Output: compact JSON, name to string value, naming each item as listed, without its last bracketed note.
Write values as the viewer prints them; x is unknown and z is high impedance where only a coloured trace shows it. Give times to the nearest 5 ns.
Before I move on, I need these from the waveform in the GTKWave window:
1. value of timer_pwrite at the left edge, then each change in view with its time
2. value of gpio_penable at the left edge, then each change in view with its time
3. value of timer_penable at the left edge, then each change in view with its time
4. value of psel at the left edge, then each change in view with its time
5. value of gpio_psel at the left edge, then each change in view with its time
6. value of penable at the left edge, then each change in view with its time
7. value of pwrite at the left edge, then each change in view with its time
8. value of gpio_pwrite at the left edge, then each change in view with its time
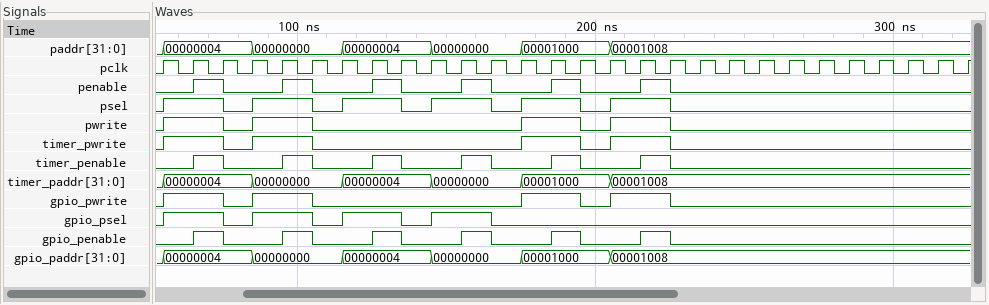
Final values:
{"value of timer_pwrite at the left edge, then each change in view with its time": "0, 1 at 55 ns, 0 at 75 ns, 1 at 85 ns, 0 at 105 ns, 1 at 175 ns, 0 at 195 ns, 1 at 205 ns, 0 at 225 ns", "value of gpio_penable at the left edge, then each change in view with its time": "0, 1 at 65 ns, 0 at 75 ns, 1 at 95 ns, 0 at 105 ns, 1 at 125 ns, 0 at 135 ns, 1 at 155 ns, 0 at 165 ns, 1 at 185 ns, 0 at 195 ns, 1 at 215 ns, 0 at 225 ns", "value of timer_penable at the left edge, then each change in view with its time": "0, 1 at 65 ns, 0 at 75 ns, 1 at 95 ns, 0 at 105 ns, 1 at 125 ns, 0 at 135 ns, 1 at 155 ns, 0 at 165 ns, 1 at 185 ns, 0 at 195 ns, 1 at 215 ns, 0 at 225 ns", "value of psel at the left edge, then each change in view with its time": "0, 1 at 55 ns, 0 at 75 ns, 1 at 85 ns, 0 at 105 ns, 1 at 115 ns, 0 at 135 ns, 1 at 145 ns, 0 at 165 ns, 1 at 175 ns, 0 at 195 ns, 1 at 205 ns, 0 at 225 ns", "value of gpio_psel at the left edge, then each change in view with its time": "0, 1 at 55 ns, 0 at 75 ns, 1 at 85 ns, 0 at 105 ns, 1 at 115 ns, 0 at 135 ns, 1 at 145 ns, 0 at 165 ns", "value of penable at the left edge, then each change in view with its time": "0, 1 at 65 ns, 0 at 75 ns, 1 at 95 ns, 0 at 105 ns, 1 at 125 ns, 0 at 135 ns, 1 at 155 ns, 0 at 165 ns, 1 at 185 ns, 0 at 195 ns, 1 at 215 ns, 0 at 225 ns", "value of pwrite at the left edge, then each change in view with its time": "0, 1 at 55 ns, 0 at 75 ns, 1 at 85 ns, 0 at 105 ns, 1 at 175 ns, 0 at 195 ns, 1 at 205 ns, 0 at 225 ns", "value of gpio_pwrite at the left edge, then each change in view with its time": "0, 1 at 55 ns, 0 at 75 ns, 1 at 85 ns, 0 at 105 ns, 1 at 175 ns, 0 at 195 ns, 1 at 205 ns, 0 at 225 ns"}
